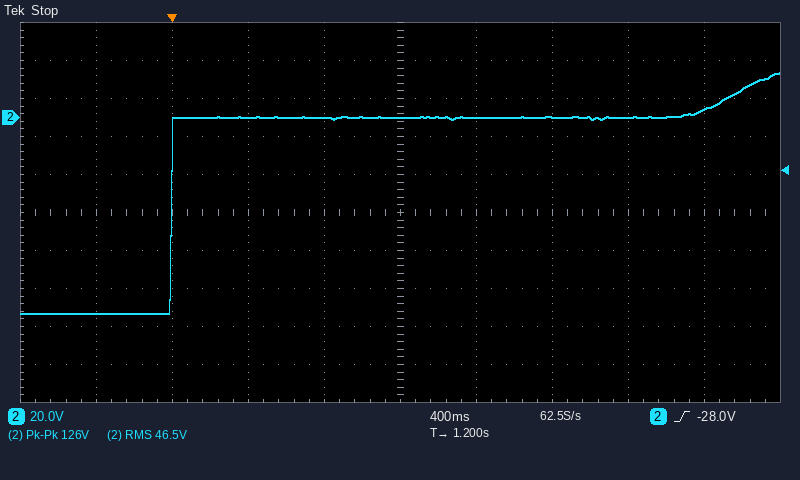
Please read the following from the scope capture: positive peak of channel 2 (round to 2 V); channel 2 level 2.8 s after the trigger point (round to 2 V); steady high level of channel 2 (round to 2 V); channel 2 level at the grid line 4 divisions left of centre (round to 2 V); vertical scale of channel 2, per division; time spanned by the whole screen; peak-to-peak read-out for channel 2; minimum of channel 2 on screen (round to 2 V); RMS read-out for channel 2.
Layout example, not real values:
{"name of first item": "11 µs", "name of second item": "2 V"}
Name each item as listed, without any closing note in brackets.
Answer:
{"positive peak of channel 2": "24 V", "channel 2 level 2.8 s after the trigger point": "4 V", "steady high level of channel 2": "0 V", "channel 2 level at the grid line 4 divisions left of centre": "-104 V", "vertical scale of channel 2, per division": "20 V", "time spanned by the whole screen": "4 s", "peak-to-peak read-out for channel 2": "126 V", "minimum of channel 2 on screen": "-104 V", "RMS read-out for channel 2": "46.5 V"}
